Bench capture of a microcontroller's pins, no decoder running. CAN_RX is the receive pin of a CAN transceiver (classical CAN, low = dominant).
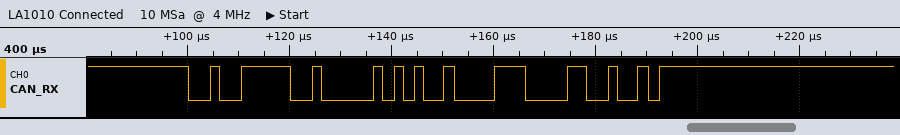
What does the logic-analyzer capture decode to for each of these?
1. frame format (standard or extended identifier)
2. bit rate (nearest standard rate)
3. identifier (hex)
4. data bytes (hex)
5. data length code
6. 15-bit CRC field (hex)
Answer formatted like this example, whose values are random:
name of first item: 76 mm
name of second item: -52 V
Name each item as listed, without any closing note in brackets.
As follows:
frame format: standard
bit rate: 500 kbit/s
identifier: 0x27D
data bytes: 48
data length code: 1
15-bit CRC field: 0x3864
